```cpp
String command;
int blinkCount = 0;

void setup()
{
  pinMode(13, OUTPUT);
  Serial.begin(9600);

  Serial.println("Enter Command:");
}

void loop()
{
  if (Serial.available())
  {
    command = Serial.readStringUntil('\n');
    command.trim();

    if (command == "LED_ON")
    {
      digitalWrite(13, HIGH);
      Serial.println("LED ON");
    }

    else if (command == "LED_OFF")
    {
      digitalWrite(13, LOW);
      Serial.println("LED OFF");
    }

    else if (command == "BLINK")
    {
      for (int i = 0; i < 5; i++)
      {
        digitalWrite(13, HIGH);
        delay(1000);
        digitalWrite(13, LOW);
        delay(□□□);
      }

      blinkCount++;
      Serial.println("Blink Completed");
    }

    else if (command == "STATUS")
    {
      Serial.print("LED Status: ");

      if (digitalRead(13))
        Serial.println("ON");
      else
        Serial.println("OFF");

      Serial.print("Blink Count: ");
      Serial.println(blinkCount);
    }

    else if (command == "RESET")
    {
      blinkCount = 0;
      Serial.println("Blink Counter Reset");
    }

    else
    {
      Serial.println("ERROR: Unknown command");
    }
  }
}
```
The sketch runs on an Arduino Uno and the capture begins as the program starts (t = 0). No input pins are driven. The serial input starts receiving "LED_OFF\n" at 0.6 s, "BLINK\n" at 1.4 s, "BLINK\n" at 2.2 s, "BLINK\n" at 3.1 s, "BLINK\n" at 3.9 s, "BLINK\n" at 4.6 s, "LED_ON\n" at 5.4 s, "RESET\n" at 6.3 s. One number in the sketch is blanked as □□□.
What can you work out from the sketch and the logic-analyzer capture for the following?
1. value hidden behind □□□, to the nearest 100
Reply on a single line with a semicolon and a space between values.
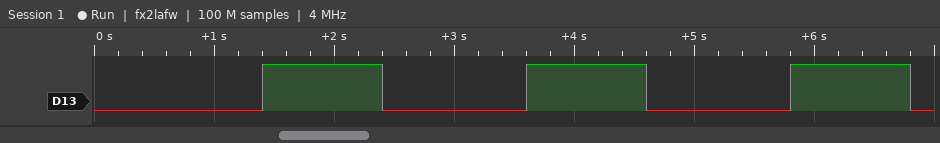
1200
